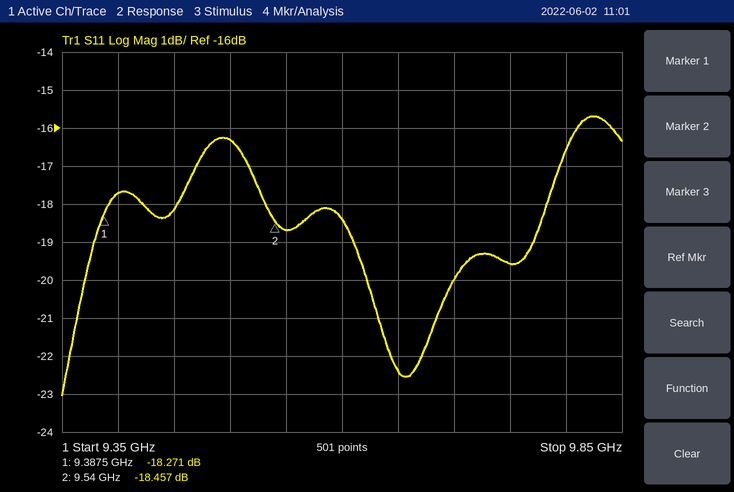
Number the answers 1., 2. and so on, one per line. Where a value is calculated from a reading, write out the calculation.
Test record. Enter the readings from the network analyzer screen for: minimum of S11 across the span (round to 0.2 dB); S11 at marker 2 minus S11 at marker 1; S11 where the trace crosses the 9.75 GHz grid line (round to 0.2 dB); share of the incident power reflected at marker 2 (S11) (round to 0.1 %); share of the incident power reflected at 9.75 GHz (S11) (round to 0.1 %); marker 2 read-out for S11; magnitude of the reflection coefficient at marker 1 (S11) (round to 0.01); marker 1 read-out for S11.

1. -23.0 dB
2. -18.457 − (-18.271) = -0.186 dB
3. -19.6 dB
4. 10^(-18.457/10) ≈ 1.4 %
5. 10^(-19.6/10) ≈ 1.1 %
6. -18.457 dB
7. 10^(-18.271/20) ≈ 0.12
8. -18.271 dB
